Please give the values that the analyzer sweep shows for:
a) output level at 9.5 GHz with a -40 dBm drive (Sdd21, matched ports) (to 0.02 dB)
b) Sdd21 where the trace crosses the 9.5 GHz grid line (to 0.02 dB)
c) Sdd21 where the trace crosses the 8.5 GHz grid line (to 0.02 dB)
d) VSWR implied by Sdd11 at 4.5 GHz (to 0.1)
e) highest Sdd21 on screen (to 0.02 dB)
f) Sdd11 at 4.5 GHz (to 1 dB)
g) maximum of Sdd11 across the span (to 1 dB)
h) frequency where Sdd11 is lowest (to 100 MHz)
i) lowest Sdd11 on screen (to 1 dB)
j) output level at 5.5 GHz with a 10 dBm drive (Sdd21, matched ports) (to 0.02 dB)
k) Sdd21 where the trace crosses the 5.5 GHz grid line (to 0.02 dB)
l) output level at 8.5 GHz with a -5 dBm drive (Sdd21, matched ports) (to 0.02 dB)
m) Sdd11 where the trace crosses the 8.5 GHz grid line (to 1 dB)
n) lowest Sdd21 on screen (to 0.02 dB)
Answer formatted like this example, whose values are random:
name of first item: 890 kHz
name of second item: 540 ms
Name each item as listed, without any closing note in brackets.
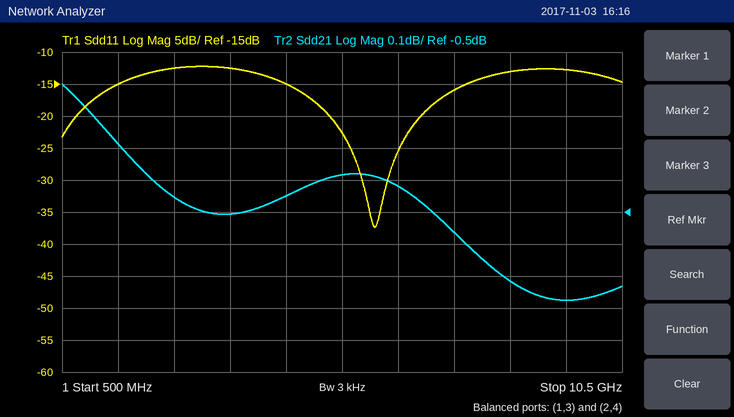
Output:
output level at 9.5 GHz with a -40 dBm drive (Sdd21, matched ports): -40.78 dBm
Sdd21 where the trace crosses the 9.5 GHz grid line: -0.78 dB
Sdd21 where the trace crosses the 8.5 GHz grid line: -0.72 dB
VSWR implied by Sdd11 at 4.5 GHz: 1.4
highest Sdd21 on screen: -0.10 dB
Sdd11 at 4.5 GHz: -15 dB
maximum of Sdd11 across the span: -12 dB
frequency where Sdd11 is lowest: 6.1 GHz
lowest Sdd11 on screen: -37 dB
output level at 5.5 GHz with a 10 dBm drive (Sdd21, matched ports): 9.62 dBm
Sdd21 where the trace crosses the 5.5 GHz grid line: -0.38 dB
output level at 8.5 GHz with a -5 dBm drive (Sdd21, matched ports): -5.72 dBm
Sdd11 where the trace crosses the 8.5 GHz grid line: -13 dB
lowest Sdd21 on screen: -0.78 dB
